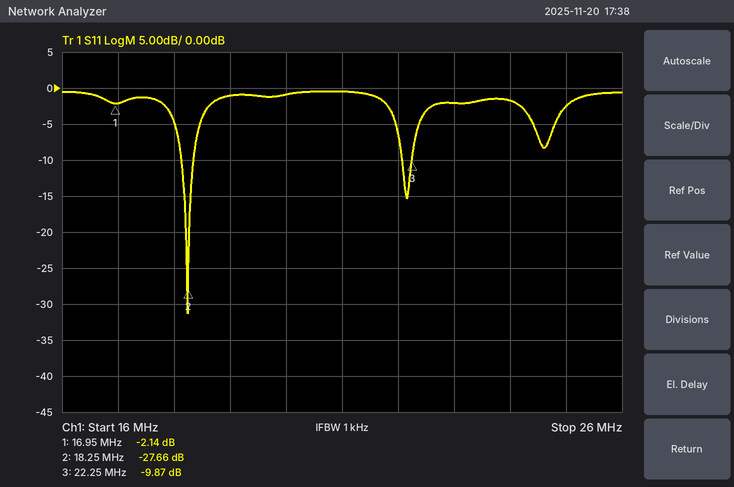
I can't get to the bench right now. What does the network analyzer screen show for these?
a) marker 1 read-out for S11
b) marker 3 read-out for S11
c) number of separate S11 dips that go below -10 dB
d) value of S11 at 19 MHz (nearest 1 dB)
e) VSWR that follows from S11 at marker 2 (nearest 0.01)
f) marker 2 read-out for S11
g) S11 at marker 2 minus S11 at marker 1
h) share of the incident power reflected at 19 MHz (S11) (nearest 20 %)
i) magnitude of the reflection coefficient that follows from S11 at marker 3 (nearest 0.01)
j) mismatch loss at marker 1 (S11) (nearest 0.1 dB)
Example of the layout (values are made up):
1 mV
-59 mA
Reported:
-2.14 dB
-9.87 dB
2
-1 dB
1.09
-27.66 dB
-25.52 dB
80 %
0.32
4.1 dB
